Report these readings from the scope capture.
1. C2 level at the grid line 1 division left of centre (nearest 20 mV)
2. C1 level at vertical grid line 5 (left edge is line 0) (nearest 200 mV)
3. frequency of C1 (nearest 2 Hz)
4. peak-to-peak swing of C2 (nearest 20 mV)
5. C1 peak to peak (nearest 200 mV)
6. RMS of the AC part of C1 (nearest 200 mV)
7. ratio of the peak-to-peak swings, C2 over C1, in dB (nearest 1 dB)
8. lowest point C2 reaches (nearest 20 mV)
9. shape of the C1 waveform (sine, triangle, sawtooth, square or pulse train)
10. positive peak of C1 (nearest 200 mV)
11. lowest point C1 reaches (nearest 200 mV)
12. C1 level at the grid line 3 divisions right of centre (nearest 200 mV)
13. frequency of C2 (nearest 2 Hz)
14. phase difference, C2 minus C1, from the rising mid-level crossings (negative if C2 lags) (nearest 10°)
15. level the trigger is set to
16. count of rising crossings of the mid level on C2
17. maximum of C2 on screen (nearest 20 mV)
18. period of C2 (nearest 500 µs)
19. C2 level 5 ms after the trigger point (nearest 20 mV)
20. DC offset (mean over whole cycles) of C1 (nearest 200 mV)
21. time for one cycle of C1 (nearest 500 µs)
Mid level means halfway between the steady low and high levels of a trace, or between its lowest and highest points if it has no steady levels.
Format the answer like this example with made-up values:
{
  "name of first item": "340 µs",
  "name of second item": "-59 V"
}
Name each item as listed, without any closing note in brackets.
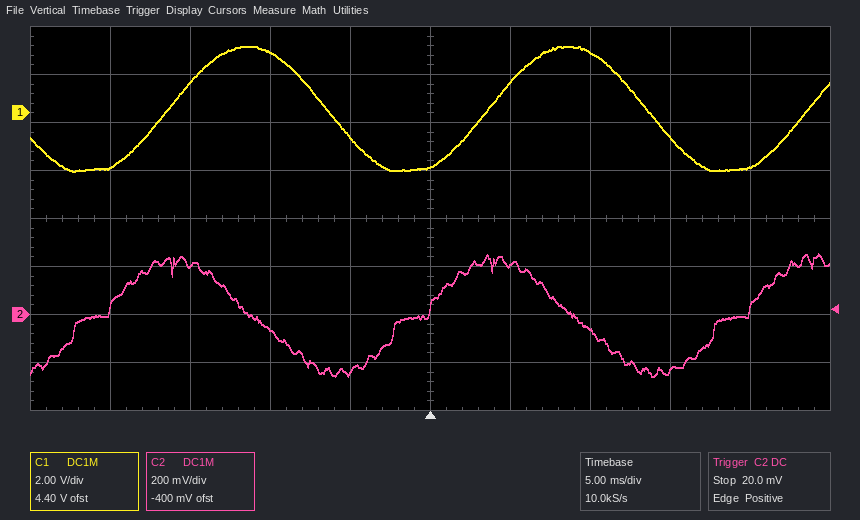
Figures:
{
  "C2 level at the grid line 1 division left of centre": "-240 mV",
  "C1 level at vertical grid line 5 (left edge is line 0)": "-2.2 V",
  "frequency of C1": "50 Hz",
  "peak-to-peak swing of C2": "520 mV",
  "C1 peak to peak": "5.2 V",
  "RMS of the AC part of C1": "1.8 V",
  "ratio of the peak-to-peak swings, C2 over C1, in dB": "-20 dB",
  "lowest point C2 reaches": "-260 mV",
  "shape of the C1 waveform": "sine",
  "positive peak of C1": "2.8 V",
  "lowest point C1 reaches": "-2.4 V",
  "C1 level at the grid line 3 divisions right of centre": "-1.0 V",
  "frequency of C2": "50 Hz",
  "phase difference, C2 minus C1, from the rising mid-level crossings (negative if C2 lags)": "+70°",
  "level the trigger is set to": "20.0 mV",
  "count of rising crossings of the mid level on C2": "3",
  "maximum of C2 on screen": "260 mV",
  "period of C2": "20.0 ms",
  "C2 level 5 ms after the trigger point": "200 mV",
  "DC offset (mean over whole cycles) of C1": "200 mV",
  "time for one cycle of C1": "20.0 ms"
}
